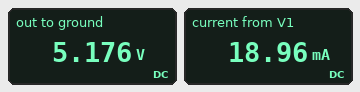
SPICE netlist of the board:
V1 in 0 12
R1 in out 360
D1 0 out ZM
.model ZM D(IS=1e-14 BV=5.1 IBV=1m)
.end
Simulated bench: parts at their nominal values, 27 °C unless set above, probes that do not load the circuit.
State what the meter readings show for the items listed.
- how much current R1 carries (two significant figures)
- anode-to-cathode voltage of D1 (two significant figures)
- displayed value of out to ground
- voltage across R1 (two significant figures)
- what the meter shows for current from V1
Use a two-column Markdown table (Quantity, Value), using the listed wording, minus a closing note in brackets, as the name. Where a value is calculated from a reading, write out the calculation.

| Quantity | Value |
|---|---|
| how much current R1 carries | (12 V - 5.176 V) / 360 Ω = 19 mA |
| anode-to-cathode voltage of D1 | 0 V - 5.176 V = -5.2 V |
| displayed value of out to ground | 5.176 V |
| voltage across R1 | 12 V - 5.176 V = 6.8 V |
| what the meter shows for current from V1 | 18.96 mA |
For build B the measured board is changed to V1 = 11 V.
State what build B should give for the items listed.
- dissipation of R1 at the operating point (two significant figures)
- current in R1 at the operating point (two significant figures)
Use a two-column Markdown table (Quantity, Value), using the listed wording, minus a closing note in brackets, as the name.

| Quantity | Value |
|---|---|
| dissipation of R1 at the operating point | 94 mW |
| current in R1 at the operating point | 16 mA |
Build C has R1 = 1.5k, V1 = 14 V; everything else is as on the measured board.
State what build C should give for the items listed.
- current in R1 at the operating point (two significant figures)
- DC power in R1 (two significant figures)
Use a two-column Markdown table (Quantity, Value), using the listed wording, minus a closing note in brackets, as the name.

| Quantity | Value |
|---|---|
| current in R1 at the operating point | 5.9 mA |
| DC power in R1 | 52 mW |
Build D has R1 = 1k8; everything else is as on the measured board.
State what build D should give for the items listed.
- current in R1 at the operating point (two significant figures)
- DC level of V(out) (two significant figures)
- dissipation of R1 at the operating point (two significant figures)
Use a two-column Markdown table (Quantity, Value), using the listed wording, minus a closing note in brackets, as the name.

| Quantity | Value |
|---|---|
| current in R1 at the operating point | 3.8 mA |
| DC level of V(out) | 5.1 V |
| dissipation of R1 at the operating point | 26 mW |
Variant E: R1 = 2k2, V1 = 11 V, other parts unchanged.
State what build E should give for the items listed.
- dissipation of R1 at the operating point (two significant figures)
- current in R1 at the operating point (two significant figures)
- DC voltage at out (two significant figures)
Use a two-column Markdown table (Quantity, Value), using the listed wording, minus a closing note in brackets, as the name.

| Quantity | Value |
|---|---|
| dissipation of R1 at the operating point | 16 mW |
| current in R1 at the operating point | 2.7 mA |
| DC voltage at out | 5.1 V |
